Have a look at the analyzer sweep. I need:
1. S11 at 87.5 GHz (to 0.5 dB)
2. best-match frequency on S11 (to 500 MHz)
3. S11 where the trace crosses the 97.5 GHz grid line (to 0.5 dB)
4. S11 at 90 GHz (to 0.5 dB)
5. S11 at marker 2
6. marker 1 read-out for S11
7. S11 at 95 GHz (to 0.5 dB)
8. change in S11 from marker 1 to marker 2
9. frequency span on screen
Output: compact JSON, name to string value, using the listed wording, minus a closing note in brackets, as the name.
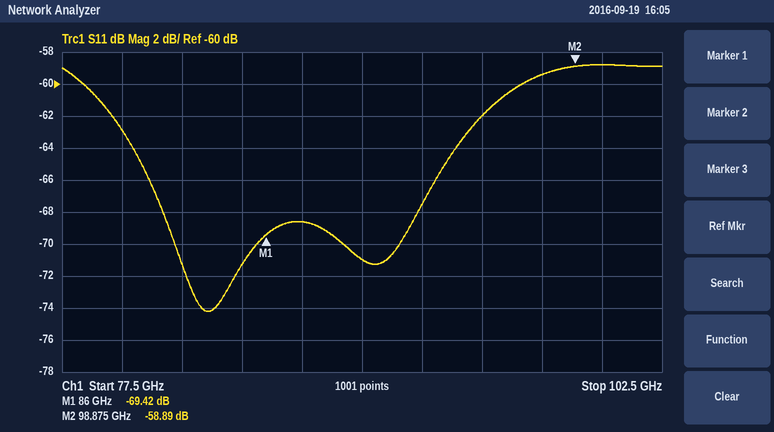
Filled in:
{"S11 at 87.5 GHz": "-68.5 dB", "best-match frequency on S11": "83.5 GHz", "S11 where the trace crosses the 97.5 GHz grid line": "-59.5 dB", "S11 at 90 GHz": "-71.0 dB", "S11 at marker 2": "-58.89 dB", "marker 1 read-out for S11": "-69.42 dB", "S11 at 95 GHz": "-62.0 dB", "change in S11 from marker 1 to marker 2": "10.53 dB", "frequency span on screen": "25 GHz"}
